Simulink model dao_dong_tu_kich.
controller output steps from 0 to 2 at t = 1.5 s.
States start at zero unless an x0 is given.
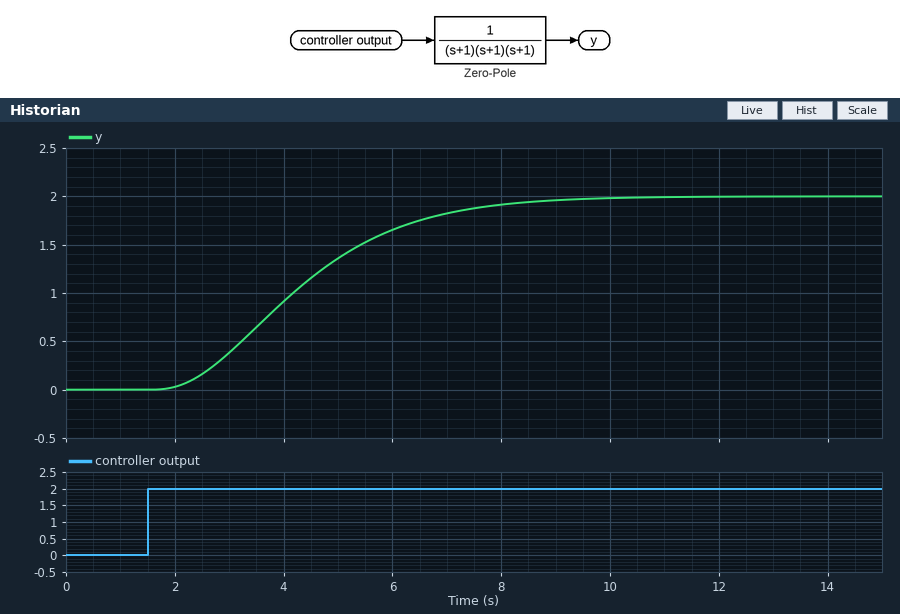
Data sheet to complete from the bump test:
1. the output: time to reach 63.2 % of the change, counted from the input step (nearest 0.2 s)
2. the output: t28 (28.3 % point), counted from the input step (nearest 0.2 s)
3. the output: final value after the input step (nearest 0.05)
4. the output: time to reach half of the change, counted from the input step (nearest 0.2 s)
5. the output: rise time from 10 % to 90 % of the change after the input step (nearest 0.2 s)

3.2 s
1.8 s
2.00
2.6 s
4.2 s
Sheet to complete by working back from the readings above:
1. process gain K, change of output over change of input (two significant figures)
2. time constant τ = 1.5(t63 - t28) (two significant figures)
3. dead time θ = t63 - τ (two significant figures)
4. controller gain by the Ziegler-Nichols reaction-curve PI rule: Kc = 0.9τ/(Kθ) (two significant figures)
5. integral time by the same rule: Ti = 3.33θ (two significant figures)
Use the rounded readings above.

1.0
2.1 s
1.1 s
1.7
3.7 s
